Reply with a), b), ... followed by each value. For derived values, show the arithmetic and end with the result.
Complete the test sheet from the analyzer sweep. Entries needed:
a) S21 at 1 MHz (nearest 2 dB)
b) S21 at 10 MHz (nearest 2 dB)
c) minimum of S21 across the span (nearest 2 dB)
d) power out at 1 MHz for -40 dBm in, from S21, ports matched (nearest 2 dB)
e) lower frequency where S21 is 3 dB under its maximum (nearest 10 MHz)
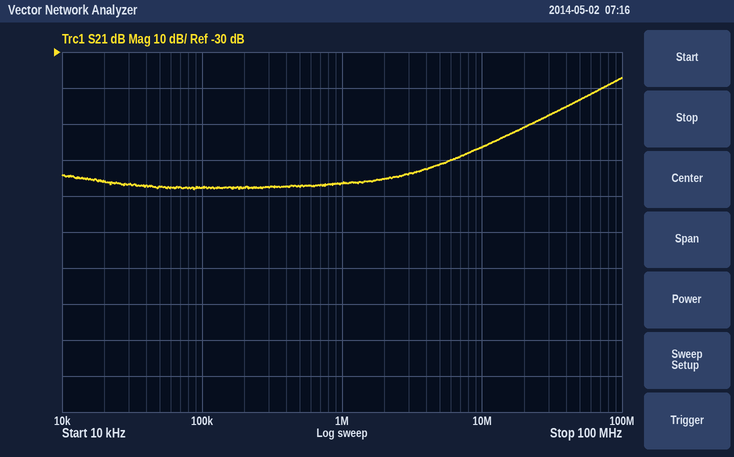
a) -66 dB
b) -56 dB
c) -68 dB
d) -40 dBm + (-66 dB) = -106 dBm
e) 70 MHz
